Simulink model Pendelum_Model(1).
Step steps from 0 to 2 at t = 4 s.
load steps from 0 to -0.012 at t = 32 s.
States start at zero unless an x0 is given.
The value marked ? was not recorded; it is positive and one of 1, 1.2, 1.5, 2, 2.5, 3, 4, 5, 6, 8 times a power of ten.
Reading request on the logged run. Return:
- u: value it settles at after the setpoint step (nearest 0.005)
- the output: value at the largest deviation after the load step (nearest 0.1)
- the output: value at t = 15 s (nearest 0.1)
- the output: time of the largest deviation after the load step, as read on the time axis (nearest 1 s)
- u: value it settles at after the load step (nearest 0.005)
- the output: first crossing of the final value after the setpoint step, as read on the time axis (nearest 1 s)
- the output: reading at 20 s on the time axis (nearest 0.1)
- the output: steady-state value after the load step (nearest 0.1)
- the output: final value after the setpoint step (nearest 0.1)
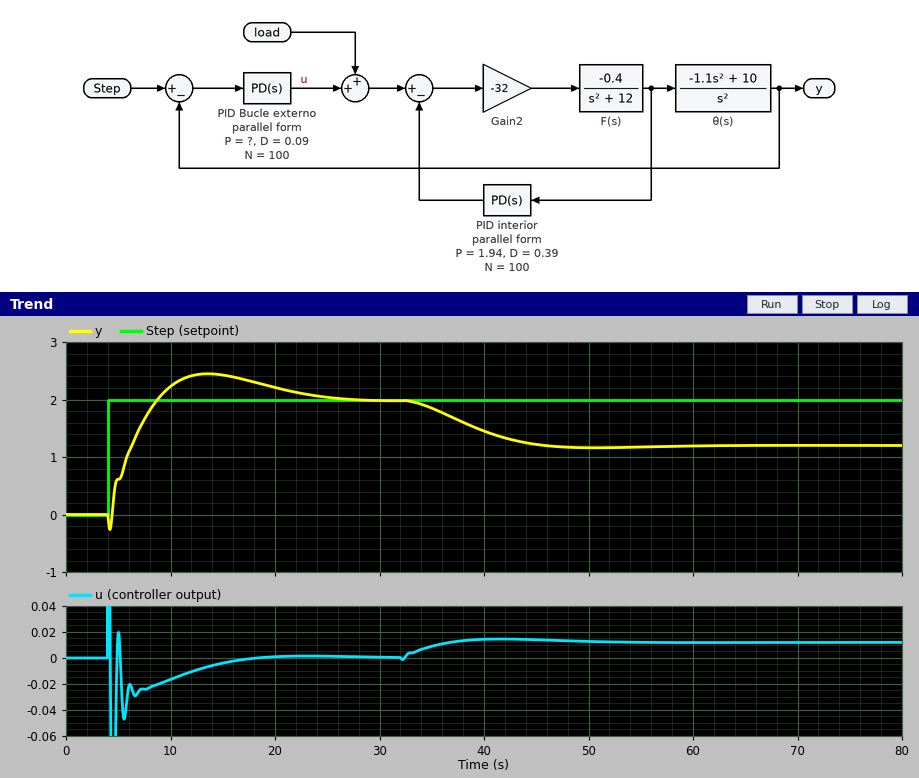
0.000
1.2
2.4
51 s
0.010
9 s
2.2
1.2
2.0
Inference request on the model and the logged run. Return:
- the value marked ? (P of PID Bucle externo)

0.015
